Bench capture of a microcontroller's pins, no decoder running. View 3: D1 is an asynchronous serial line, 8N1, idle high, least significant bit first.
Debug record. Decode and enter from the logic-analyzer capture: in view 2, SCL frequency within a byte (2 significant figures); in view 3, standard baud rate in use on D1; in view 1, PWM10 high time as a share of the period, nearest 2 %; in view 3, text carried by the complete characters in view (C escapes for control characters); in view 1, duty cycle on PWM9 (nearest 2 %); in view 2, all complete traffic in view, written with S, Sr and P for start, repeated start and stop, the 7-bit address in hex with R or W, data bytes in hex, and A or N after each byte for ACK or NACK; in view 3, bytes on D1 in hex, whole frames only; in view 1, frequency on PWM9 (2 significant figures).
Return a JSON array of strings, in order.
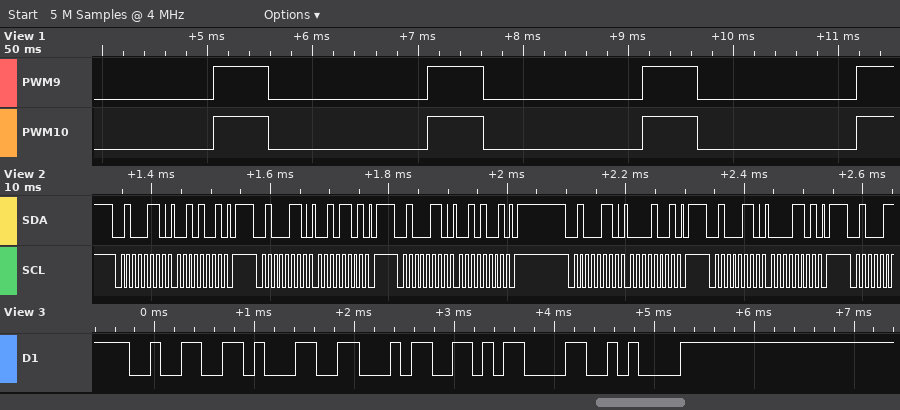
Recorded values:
["100 kHz", "9600 baud", "26 %", "\"214\\r\\n\"", "26 %", "S 23W A 29 A P S 23W A 2D A P S 23W A 29 A P S 23W A 09 A P S 23W A 0D A P", "32 31 34 0D 0A", "490 Hz"]
